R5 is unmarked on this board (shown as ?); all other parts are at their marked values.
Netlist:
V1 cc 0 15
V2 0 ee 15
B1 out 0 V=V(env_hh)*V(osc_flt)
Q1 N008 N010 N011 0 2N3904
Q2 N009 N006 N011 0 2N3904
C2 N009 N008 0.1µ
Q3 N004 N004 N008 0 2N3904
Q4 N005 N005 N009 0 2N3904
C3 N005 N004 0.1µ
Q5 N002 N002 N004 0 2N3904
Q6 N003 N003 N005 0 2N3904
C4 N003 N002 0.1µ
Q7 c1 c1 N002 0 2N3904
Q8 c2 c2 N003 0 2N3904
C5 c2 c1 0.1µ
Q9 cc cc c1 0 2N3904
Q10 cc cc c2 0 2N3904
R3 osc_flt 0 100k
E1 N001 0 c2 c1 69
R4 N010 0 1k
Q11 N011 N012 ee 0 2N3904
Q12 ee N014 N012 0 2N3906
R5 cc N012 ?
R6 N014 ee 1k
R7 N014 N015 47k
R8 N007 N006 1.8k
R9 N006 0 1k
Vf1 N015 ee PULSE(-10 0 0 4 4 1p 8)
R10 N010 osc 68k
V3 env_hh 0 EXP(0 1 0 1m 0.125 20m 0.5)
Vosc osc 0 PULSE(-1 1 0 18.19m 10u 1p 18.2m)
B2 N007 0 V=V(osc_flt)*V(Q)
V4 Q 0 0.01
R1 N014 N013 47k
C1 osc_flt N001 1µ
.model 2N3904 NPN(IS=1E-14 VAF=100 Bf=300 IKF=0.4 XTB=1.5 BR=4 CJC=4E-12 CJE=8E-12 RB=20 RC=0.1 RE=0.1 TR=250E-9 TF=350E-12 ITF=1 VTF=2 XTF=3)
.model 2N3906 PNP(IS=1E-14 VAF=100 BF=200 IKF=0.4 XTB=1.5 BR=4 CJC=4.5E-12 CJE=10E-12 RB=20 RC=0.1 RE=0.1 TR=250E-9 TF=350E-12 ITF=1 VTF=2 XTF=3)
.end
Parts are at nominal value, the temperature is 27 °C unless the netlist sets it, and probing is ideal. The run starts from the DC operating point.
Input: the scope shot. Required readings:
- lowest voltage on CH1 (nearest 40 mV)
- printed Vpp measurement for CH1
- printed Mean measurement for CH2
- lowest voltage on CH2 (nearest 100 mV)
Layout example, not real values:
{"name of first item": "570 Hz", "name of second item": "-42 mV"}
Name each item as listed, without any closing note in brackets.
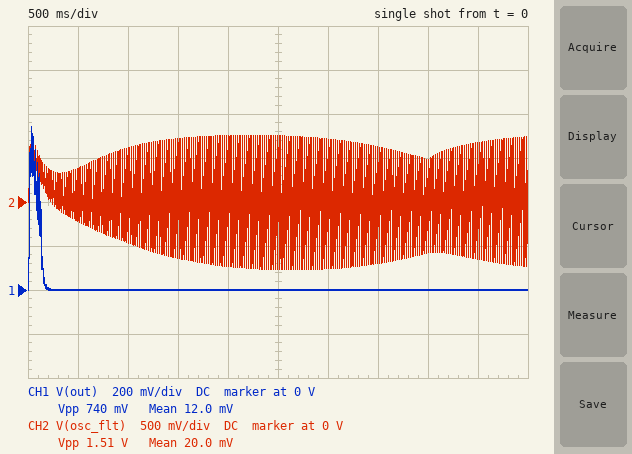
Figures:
{"lowest voltage on CH1": "0 V", "printed Vpp measurement for CH1": "740 mV", "printed Mean measurement for CH2": "20.0 mV", "lowest voltage on CH2": "-800 mV"}
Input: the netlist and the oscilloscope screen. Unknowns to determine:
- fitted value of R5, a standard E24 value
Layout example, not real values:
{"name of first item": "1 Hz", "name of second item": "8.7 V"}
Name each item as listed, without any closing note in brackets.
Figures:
{"fitted value of R5, a standard E24 value": "5.6 kΩ"}
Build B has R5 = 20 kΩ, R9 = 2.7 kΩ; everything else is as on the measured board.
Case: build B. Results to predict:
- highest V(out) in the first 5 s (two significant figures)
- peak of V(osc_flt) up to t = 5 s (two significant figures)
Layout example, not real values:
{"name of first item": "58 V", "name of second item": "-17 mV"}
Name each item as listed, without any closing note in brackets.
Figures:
{"highest V(out) in the first 5 s": "330 mV", "peak of V(osc_flt) up to t = 5 s": "670 mV"}
